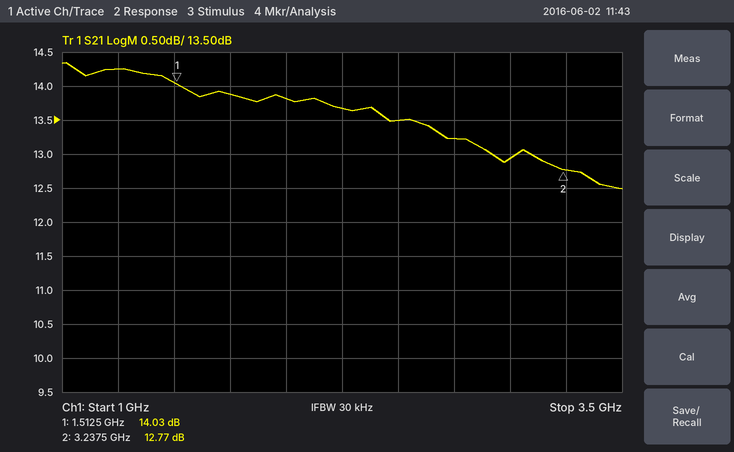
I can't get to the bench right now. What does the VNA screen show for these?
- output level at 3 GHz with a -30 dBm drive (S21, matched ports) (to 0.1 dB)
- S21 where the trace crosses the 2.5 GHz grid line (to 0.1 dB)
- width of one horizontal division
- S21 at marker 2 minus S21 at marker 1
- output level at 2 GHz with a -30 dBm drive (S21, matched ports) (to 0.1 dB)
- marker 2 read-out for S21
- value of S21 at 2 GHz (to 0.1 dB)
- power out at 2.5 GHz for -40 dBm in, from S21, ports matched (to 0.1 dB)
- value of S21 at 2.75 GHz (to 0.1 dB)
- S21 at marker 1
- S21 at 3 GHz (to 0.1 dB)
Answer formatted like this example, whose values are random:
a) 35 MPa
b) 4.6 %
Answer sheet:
a) -17.1 dBm
b) 13.5 dB
c) 250 MHz
d) -1.26 dB
e) -16.2 dBm
f) 12.77 dB
g) 13.8 dB
h) -26.5 dBm
i) 13.2 dB
j) 14.03 dB
k) 12.9 dB
